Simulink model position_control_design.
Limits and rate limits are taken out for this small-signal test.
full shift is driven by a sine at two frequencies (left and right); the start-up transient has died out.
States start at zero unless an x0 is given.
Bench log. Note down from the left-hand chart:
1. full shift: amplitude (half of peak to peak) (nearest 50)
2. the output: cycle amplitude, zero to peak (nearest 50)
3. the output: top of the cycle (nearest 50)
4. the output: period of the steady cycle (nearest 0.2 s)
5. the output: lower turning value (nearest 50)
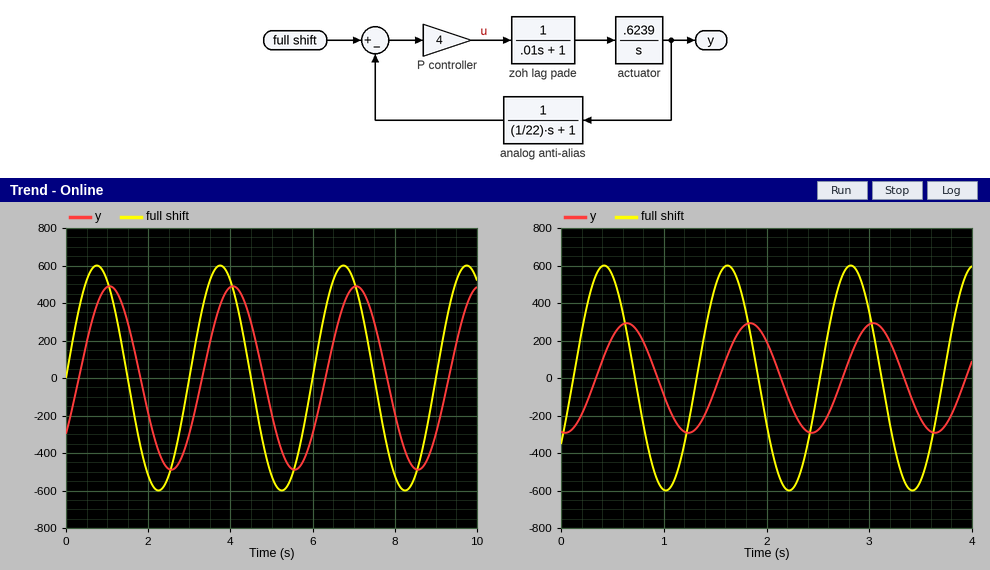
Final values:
600
500
500
3.0 s
-500
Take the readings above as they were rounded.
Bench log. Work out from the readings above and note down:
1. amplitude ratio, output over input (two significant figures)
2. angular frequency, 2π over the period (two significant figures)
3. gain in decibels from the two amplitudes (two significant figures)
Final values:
0.83
2.1 rad/s
-1.6 dB
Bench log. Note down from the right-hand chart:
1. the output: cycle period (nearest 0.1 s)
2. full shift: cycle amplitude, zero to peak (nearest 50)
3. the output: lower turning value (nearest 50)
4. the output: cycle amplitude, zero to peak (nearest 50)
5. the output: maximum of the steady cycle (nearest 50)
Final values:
1.2 s
600
-300
300
300
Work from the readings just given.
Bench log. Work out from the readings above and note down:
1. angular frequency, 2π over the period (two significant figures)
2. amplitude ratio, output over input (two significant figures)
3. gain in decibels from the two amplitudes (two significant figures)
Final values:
5.2 rad/s
0.50
-6.0 dB
